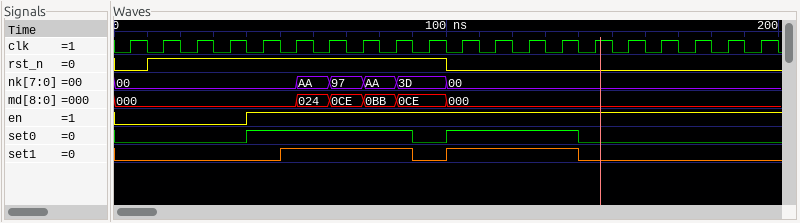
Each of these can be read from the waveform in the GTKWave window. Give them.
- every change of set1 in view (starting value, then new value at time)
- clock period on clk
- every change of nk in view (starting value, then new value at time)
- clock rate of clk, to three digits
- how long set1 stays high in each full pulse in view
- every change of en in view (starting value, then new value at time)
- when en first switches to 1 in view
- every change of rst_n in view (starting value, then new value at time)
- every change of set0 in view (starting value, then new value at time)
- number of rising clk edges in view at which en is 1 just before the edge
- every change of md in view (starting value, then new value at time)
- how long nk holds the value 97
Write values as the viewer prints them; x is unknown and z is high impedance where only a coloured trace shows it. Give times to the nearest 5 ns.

0, 1 at 50 ns, 0 at 90 ns, 1 at 100 ns, 0 at 140 ns
10 ns
00, AA at 55 ns, 97 at 65 ns, AA at 75 ns, 3D at 85 ns, 00 at 100 ns
100 MHz
40 ns, 40 ns
0, 1 at 40 ns
40 ns
0, 1 at 10 ns, 0 at 100 ns
0, 1 at 40 ns, 0 at 90 ns, 1 at 100 ns, 0 at 140 ns
16
000, 024 at 55 ns, 0CE at 65 ns, 0BB at 75 ns, 0CE at 85 ns, 000 at 100 ns
10 ns
